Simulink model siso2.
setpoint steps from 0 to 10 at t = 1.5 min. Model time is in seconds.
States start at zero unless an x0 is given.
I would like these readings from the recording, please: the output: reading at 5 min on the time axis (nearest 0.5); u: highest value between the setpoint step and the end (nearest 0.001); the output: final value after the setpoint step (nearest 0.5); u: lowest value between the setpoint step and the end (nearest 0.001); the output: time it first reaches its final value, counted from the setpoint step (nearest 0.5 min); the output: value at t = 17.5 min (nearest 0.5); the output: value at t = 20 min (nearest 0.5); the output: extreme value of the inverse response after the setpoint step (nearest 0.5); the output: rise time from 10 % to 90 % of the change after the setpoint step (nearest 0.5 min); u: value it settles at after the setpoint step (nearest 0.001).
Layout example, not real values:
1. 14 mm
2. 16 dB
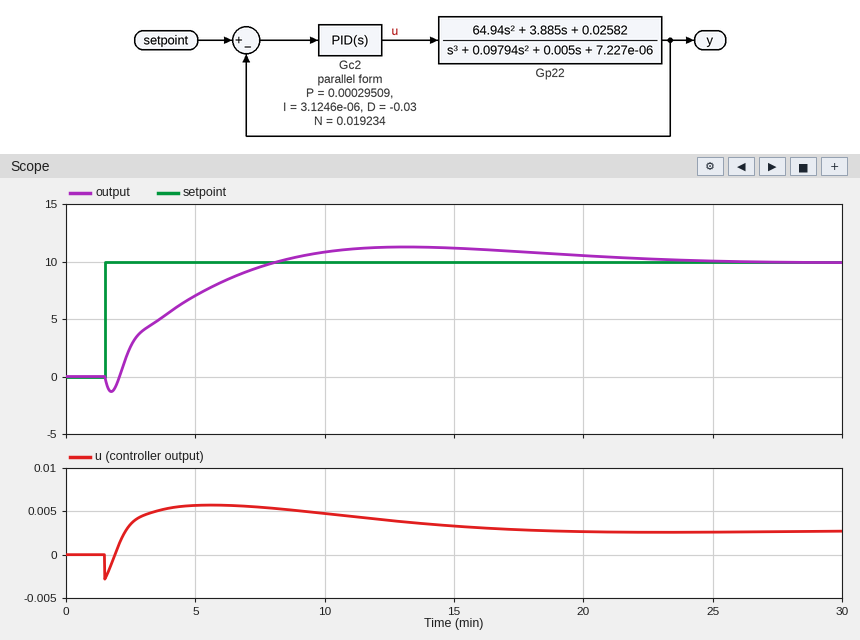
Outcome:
1. 7.0
2. 0.006
3. 10.0
4. -0.003
5. 6.5 min
6. 11.0
7. 10.5
8. -1.5
9. 4.5 min
10. 0.003
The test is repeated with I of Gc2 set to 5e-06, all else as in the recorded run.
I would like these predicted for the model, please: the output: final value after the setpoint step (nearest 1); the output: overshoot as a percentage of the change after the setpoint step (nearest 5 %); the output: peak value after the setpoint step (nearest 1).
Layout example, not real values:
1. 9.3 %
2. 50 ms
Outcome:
1. 10
2. 15 %
3. 11
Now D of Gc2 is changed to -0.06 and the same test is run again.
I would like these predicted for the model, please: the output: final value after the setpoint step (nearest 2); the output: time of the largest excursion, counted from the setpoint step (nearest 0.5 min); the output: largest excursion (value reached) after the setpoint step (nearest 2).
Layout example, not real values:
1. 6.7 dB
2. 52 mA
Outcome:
1. 10
2. 11.0 min
3. 12
